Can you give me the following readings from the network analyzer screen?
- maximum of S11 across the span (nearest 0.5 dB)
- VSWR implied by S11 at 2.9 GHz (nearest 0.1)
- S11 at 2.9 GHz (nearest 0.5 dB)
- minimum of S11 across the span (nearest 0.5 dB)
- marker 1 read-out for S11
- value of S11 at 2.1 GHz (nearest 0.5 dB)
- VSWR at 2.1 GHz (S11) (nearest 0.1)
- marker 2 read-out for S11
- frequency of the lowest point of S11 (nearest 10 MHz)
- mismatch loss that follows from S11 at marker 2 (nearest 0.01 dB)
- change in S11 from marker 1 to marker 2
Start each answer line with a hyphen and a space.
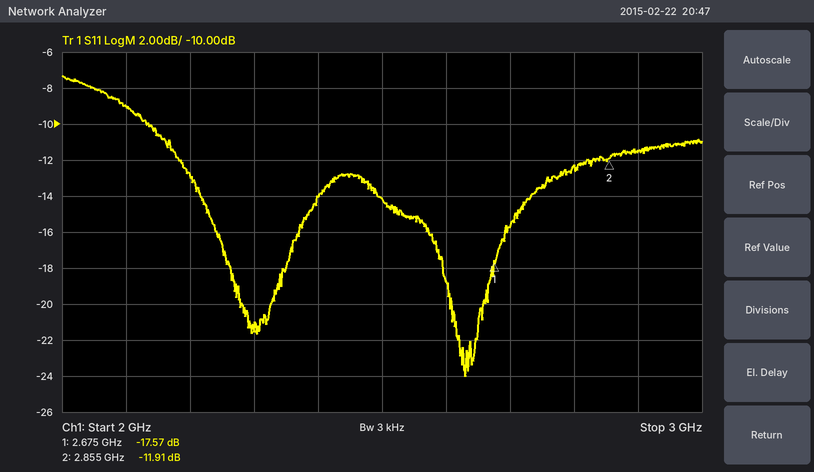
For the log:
- -7.5 dB
- 1.7
- -11.5 dB
- -24.0 dB
- -17.57 dB
- -9.0 dB
- 2.1
- -11.91 dB
- 2.63 GHz
- 0.29 dB
- 5.66 dB
